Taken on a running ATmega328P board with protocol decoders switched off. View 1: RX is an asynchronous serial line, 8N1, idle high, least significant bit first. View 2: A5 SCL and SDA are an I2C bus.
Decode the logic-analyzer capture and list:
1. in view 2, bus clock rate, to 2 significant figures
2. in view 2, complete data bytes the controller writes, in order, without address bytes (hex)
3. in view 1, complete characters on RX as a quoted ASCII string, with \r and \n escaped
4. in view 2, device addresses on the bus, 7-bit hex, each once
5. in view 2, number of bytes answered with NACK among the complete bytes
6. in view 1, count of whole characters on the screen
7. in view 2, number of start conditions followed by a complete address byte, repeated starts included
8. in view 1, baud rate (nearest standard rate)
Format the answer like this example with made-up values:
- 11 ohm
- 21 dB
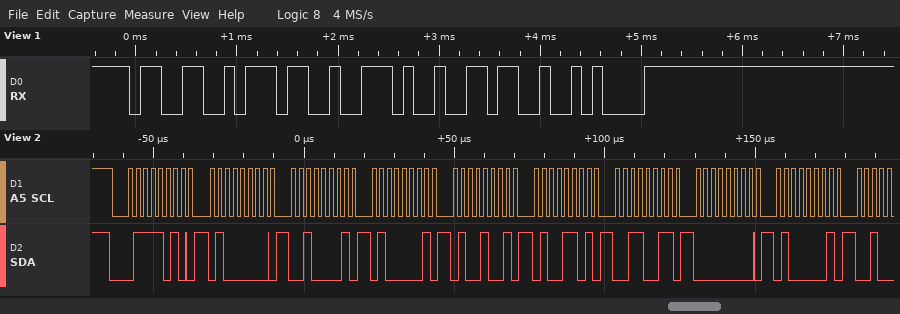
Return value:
- 400 kHz
- 40 21 41 49 4D 33 00 41
- "37.6\n"
- 0x3D
- 0
- 5
- 1
- 9600 baud
